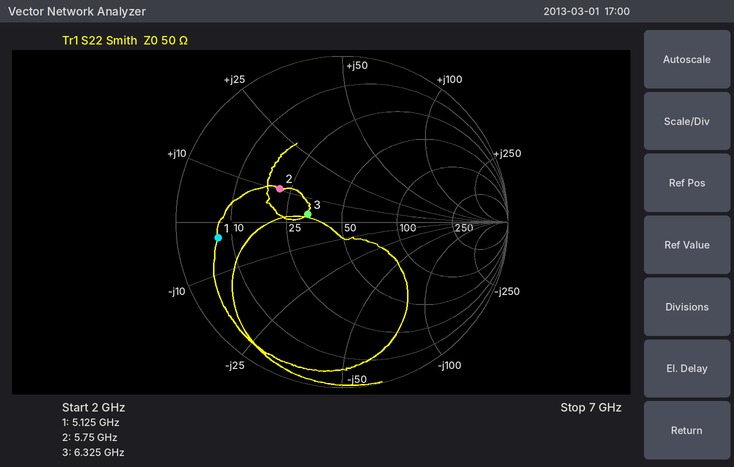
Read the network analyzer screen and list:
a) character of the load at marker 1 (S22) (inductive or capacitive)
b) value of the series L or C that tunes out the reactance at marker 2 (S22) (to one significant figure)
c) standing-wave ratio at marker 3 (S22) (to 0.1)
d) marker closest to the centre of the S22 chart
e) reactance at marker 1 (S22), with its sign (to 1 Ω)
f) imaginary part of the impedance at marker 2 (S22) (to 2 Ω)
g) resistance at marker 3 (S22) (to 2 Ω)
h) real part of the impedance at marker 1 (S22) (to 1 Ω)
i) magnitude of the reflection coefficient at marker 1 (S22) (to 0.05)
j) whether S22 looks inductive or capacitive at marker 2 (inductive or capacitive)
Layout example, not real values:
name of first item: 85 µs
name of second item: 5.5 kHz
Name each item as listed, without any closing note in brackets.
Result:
character of the load at marker 1 (S22): capacitive
value of the series L or C that tunes out the reactance at marker 2 (S22): 3 pF
standing-wave ratio at marker 3 (S22): 1.5
marker closest to the centre of the S22 chart: marker 3
reactance at marker 1 (S22), with its sign: -3 Ω
imaginary part of the impedance at marker 2 (S22): +10 Ω
resistance at marker 3 (S22): 32 Ω
real part of the impedance at marker 1 (S22): 7 Ω
magnitude of the reflection coefficient at marker 1 (S22): 0.75
whether S22 looks inductive or capacitive at marker 2: inductive
